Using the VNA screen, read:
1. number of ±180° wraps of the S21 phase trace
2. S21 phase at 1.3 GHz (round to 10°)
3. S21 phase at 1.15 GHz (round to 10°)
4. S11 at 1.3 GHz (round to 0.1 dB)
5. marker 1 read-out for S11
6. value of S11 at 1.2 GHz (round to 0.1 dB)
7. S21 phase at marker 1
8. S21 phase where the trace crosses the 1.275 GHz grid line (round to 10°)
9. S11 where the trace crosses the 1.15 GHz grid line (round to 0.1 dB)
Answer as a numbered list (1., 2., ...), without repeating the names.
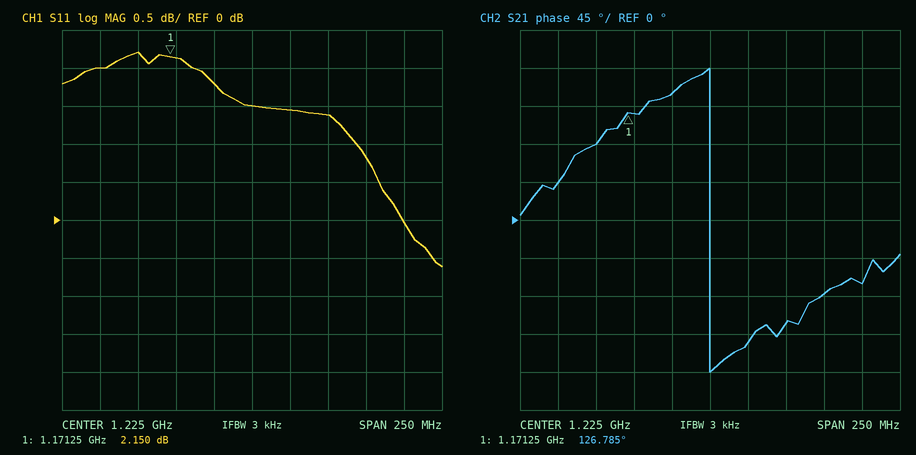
1. 1
2. -90°
3. 90°
4. 0.8 dB
5. 2.150 dB
6. 1.8 dB
7. 126.785°
8. -120°
9. 2.2 dB
